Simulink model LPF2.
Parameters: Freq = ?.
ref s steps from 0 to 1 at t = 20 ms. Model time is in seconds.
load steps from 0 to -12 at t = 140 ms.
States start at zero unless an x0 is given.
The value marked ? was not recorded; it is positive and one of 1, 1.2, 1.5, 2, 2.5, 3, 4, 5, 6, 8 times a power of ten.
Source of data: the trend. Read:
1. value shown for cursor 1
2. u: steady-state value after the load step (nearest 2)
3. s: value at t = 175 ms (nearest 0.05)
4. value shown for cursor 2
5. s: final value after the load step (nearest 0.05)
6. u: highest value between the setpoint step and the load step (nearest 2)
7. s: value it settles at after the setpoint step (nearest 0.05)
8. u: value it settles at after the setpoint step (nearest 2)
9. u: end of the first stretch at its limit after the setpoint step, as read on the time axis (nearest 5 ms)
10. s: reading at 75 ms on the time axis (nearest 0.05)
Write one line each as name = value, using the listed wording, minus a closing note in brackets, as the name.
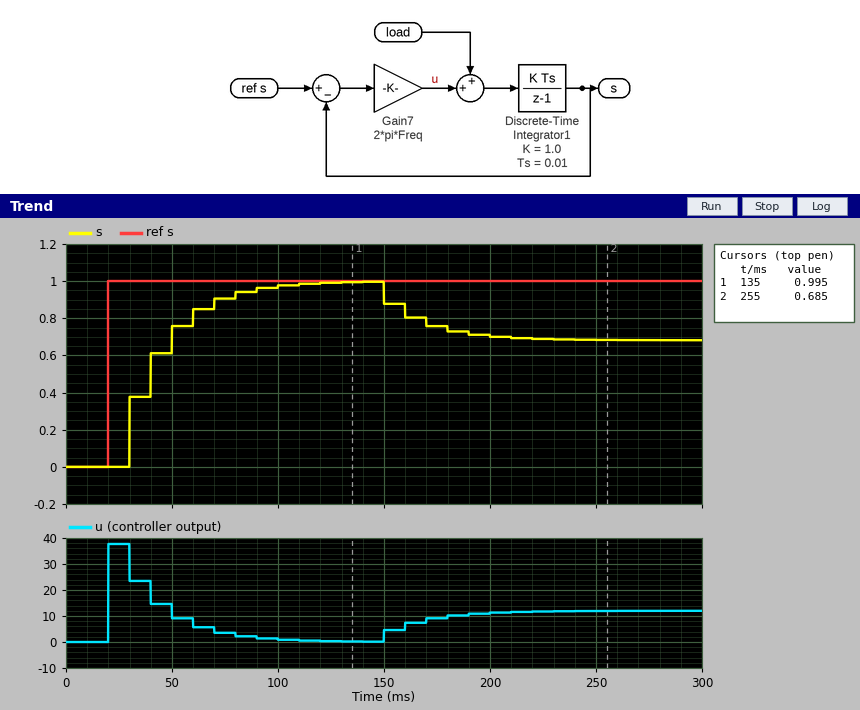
value shown for cursor 1 = 0.995
u: steady-state value after the load step = 12
s: value at t = 175 ms = 0.75
value shown for cursor 2 = 0.685
s: final value after the load step = 0.70
u: highest value between the setpoint step and the load step = 38
s: value it settles at after the setpoint step = 1.00
u: value it settles at after the setpoint step = 0
u: end of the first stretch at its limit after the setpoint step, as read on the time axis = 30 ms
s: reading at 75 ms on the time axis = 0.90
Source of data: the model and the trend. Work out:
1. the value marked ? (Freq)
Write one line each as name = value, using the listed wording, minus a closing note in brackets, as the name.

the value marked ? = 6
